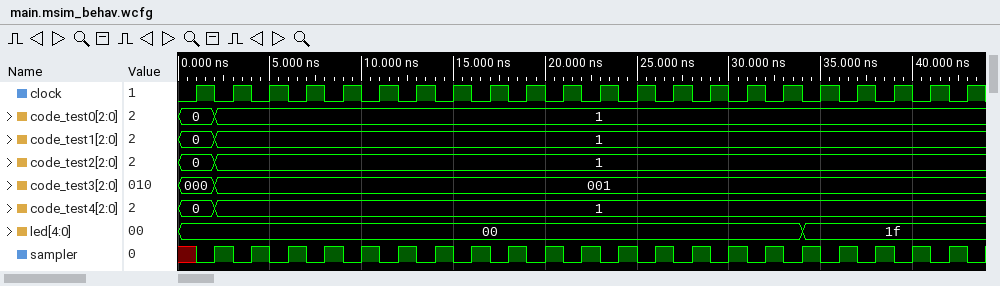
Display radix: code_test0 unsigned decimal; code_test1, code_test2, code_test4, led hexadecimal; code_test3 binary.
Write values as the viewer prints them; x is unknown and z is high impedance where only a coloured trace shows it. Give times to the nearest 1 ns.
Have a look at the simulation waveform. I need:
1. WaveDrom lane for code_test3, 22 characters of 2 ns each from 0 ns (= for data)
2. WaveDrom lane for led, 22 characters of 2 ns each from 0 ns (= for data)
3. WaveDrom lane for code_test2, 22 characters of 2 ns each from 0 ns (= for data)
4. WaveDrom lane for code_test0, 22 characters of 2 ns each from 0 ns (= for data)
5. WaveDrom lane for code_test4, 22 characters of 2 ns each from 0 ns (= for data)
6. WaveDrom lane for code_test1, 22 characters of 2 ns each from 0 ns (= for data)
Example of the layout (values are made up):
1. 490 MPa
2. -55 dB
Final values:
1. {name: 'code_test3', wave: '==....................', data: '000 001'}
2. {name: 'led', wave: '=................=....', data: '00 1f'}
3. {name: 'code_test2', wave: '==....................', data: '0 1'}
4. {name: 'code_test0', wave: '==....................', data: '0 1'}
5. {name: 'code_test4', wave: '==....................', data: '0 1'}
6. {name: 'code_test1', wave: '==....................', data: '0 1'}
